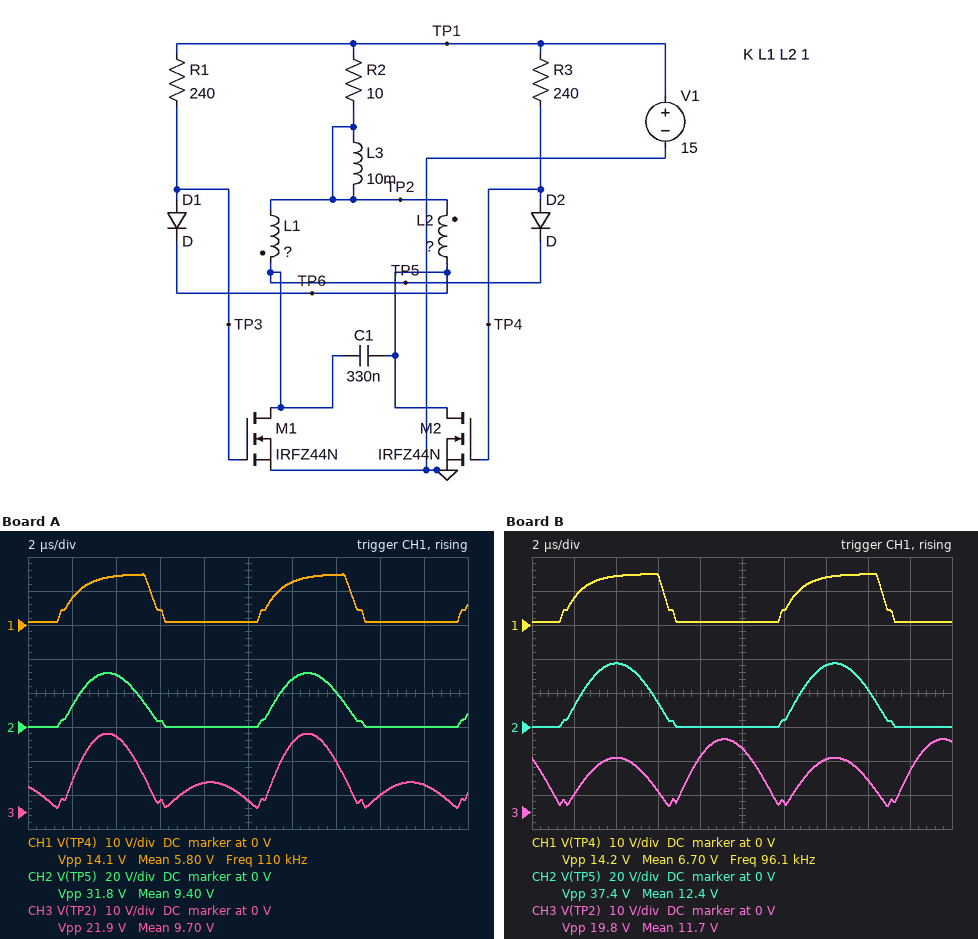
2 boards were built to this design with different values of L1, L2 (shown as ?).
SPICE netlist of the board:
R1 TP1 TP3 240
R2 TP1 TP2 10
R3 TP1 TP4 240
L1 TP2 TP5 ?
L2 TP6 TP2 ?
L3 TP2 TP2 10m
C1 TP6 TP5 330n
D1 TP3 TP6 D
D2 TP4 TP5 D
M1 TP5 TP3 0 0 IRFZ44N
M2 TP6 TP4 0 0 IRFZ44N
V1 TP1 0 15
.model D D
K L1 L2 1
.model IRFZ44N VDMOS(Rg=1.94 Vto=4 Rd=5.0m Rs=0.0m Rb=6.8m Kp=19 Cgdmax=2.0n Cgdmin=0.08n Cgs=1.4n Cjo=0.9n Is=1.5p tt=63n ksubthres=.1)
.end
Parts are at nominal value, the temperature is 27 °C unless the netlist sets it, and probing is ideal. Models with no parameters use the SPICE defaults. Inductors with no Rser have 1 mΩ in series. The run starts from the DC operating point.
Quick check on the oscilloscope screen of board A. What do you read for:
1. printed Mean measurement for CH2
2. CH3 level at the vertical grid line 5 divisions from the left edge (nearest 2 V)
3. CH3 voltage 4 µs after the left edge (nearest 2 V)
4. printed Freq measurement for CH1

9.40 V
4 V
22 V
110 kHz
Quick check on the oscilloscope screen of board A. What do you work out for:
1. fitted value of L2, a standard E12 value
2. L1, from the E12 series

3.3 µH
470 nH
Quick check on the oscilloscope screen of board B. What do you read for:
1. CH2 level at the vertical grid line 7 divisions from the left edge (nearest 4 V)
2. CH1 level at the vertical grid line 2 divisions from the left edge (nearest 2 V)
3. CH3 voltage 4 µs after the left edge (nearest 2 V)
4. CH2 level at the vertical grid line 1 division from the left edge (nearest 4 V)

36 V
14 V
16 V
12 V
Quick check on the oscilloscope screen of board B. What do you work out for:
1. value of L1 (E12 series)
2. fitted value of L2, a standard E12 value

2.7 µH
1.5 µH
